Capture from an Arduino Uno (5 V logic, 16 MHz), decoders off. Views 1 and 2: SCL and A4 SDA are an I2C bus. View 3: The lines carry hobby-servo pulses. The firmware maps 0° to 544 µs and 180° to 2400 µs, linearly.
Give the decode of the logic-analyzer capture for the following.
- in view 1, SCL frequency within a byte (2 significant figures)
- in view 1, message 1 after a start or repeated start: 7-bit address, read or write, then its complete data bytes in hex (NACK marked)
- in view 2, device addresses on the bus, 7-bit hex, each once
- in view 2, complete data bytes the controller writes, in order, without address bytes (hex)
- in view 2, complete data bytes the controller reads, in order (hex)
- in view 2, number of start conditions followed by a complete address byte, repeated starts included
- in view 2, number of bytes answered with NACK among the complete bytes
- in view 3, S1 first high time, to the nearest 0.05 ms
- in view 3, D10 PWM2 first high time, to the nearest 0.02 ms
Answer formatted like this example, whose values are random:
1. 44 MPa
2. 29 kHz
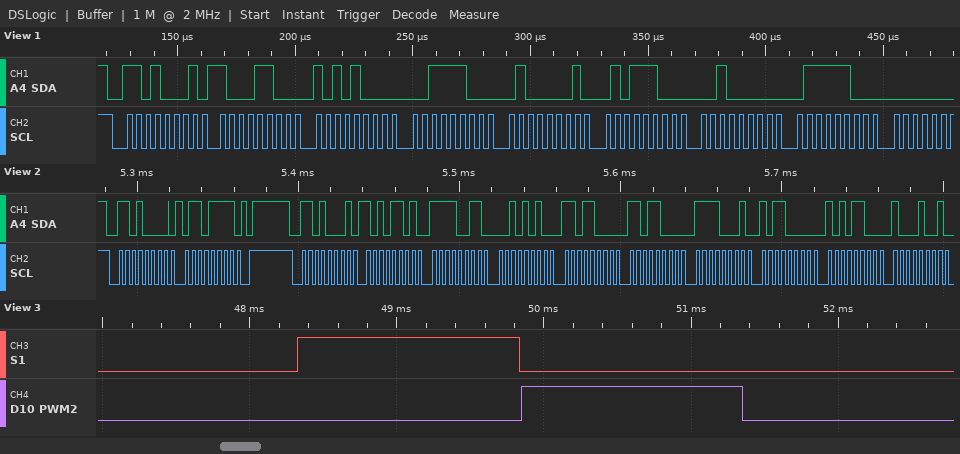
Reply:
1. 250 kHz
2. 0x68 read: 8C A8 3C 41 5C 20 7C
3. 0x68
4. 6F
5. AD F3 2A D8 D8 F1 B0 AC 89
6. 2
7. 0
8. 1.50 ms
9. 1.50 ms
